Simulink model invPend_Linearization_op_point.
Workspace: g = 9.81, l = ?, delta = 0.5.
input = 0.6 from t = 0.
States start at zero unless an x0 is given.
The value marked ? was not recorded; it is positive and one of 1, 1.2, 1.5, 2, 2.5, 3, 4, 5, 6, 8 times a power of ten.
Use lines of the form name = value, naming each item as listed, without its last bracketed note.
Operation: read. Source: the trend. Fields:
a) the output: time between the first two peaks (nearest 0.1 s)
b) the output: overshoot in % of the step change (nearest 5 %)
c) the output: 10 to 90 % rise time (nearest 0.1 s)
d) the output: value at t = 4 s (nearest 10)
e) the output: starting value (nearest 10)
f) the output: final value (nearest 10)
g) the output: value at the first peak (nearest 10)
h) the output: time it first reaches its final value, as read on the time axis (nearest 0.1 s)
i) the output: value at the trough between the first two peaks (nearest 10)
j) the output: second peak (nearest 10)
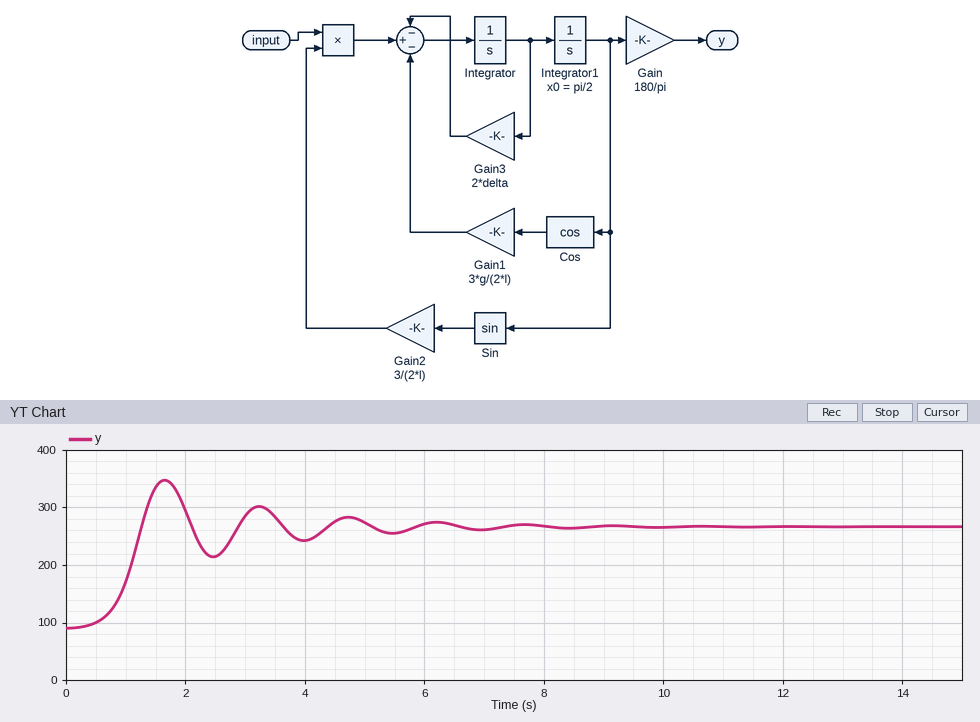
the output: time between the first two peaks = 1.6 s
the output: overshoot in % of the step change = 45 %
the output: 10 to 90 % rise time = 0.6 s
the output: value at t = 4 s = 240
the output: starting value = 90
the output: final value = 270
the output: value at the first peak = 350
the output: time it first reaches its final value, as read on the time axis = 1.3 s
the output: value at the trough between the first two peaks = 210
the output: second peak = 300
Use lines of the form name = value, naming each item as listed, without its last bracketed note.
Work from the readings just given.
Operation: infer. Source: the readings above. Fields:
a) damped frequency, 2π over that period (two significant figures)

damped frequency, 2π over that period = 3.9 rad/s
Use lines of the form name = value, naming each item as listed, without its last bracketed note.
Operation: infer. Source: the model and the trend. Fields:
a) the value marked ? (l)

the value marked ? = 0.8
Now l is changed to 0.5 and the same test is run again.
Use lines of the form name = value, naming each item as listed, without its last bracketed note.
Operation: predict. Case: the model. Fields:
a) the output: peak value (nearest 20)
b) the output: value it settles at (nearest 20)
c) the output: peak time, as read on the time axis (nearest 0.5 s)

the output: peak value = 360
the output: value it settles at = 260
the output: peak time, as read on the time axis = 1.5 s
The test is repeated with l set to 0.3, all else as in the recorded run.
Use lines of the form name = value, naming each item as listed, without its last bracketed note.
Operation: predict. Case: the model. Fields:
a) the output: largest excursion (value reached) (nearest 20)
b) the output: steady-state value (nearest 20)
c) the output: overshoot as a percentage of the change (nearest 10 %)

the output: largest excursion (value reached) = 360
the output: steady-state value = 260
the output: overshoot as a percentage of the change = 60 %
